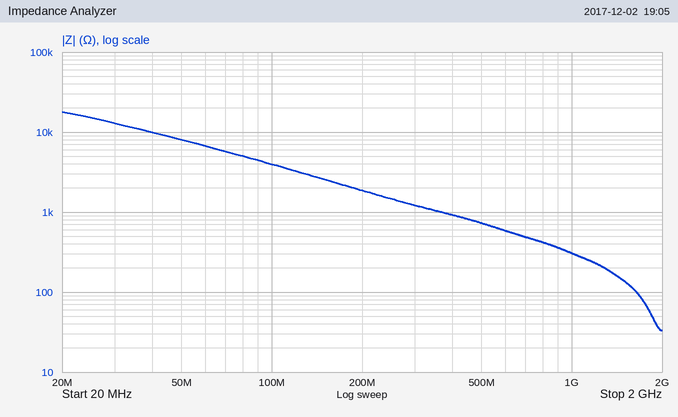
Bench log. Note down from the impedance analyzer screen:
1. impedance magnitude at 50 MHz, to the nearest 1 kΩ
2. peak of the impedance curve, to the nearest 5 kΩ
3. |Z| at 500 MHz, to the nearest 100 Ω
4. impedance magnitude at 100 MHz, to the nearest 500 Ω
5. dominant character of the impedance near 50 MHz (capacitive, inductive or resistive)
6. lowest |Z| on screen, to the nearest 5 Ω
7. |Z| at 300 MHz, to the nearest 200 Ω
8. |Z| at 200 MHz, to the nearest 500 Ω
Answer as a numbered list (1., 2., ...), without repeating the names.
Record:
1. 8 kΩ
2. 20 kΩ
3. 700 Ω
4. 4.0 kΩ
5. capacitive
6. 35 Ω
7. 1.2 kΩ
8. 2.0 kΩ
